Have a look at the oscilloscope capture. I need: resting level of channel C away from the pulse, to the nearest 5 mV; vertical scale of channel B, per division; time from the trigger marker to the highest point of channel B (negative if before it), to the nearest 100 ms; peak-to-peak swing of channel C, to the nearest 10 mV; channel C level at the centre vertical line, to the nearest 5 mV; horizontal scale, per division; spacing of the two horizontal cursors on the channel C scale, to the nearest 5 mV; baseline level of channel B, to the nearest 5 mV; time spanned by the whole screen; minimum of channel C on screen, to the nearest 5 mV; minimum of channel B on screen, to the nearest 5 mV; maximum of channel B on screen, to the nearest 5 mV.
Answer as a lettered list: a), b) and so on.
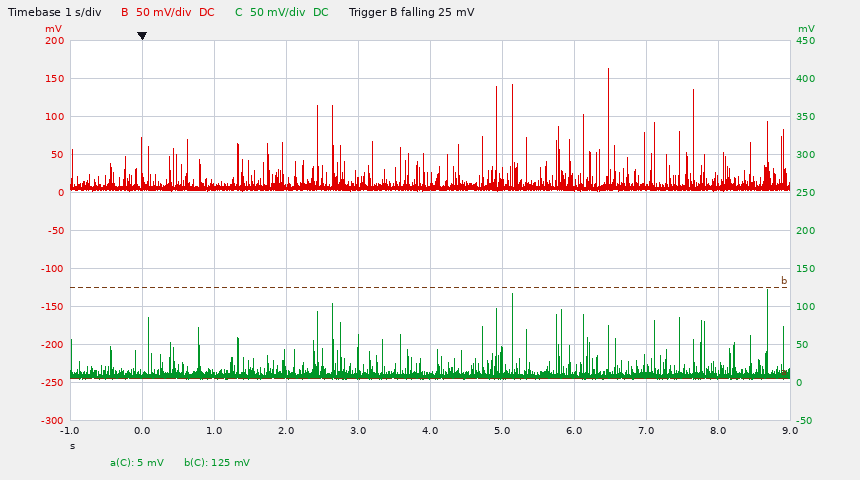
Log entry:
a) 10 mV
b) 50 mV
c) +6.5 s
d) 120 mV
e) 10 mV
f) 1 s
g) 120 mV
h) 5 mV
i) 10 s
j) 5 mV
k) 0 mV
l) 165 mV
